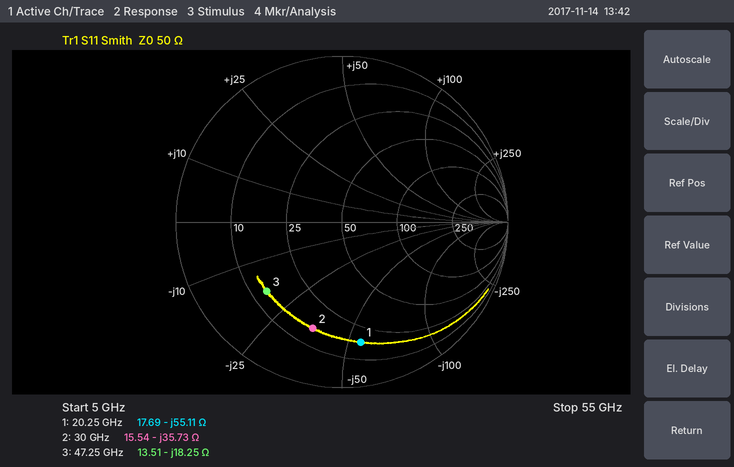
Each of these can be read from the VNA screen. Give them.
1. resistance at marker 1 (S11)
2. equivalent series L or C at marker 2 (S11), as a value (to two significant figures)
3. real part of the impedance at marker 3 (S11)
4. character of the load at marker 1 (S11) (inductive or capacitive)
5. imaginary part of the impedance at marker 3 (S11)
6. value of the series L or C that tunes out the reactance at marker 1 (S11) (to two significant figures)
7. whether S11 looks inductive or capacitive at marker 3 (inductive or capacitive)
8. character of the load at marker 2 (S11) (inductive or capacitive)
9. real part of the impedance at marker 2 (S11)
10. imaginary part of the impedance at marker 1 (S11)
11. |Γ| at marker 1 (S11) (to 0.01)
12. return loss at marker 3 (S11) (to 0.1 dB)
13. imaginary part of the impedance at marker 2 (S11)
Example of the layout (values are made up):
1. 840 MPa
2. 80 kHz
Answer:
1. 17.69 Ω
2. 150 fF
3. 13.51 Ω
4. capacitive
5. -18.25 Ω
6. 430 pH
7. capacitive
8. capacitive
9. 15.54 Ω
10. -55.11 Ω
11. 0.73
12. 4.2 dB
13. -35.73 Ω
